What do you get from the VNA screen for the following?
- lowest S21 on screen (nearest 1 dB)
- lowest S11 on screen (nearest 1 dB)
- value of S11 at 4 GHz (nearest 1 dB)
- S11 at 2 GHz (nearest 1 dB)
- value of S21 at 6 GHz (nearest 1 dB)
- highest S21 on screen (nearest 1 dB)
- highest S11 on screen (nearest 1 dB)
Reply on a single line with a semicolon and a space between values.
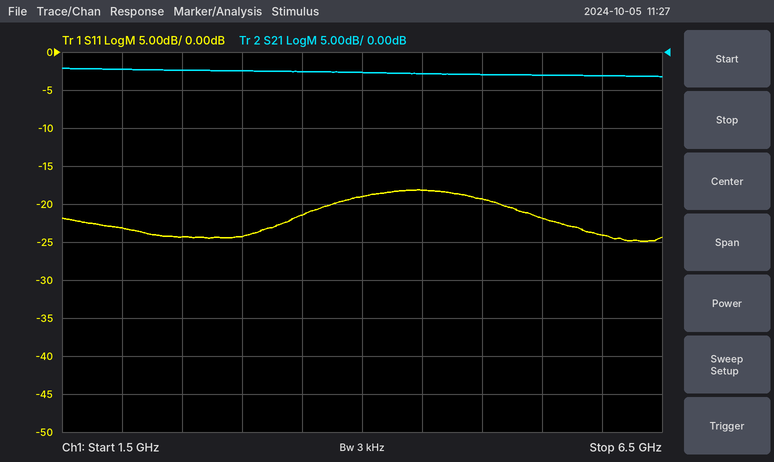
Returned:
-3 dB; -25 dB; -19 dB; -23 dB; -3 dB; -2 dB; -18 dB
